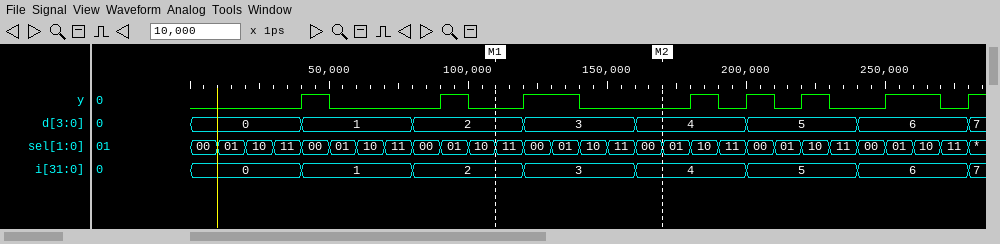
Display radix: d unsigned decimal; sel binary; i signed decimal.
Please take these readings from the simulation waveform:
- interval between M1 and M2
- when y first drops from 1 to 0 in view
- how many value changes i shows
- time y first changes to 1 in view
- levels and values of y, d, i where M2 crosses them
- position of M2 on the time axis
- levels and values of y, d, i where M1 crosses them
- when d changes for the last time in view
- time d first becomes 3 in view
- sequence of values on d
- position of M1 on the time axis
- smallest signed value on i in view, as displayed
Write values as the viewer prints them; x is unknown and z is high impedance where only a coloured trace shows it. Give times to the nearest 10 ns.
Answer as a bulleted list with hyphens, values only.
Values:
- 60 ns
- 50 ns
- 7
- 40 ns
- y=0, d=4, i=4
- 170 ns
- y=0, d=2, i=2
- 280 ns
- 120 ns
- 0, 1, 2, 3, 4, 5, 6, 7
- 110 ns
- 0
